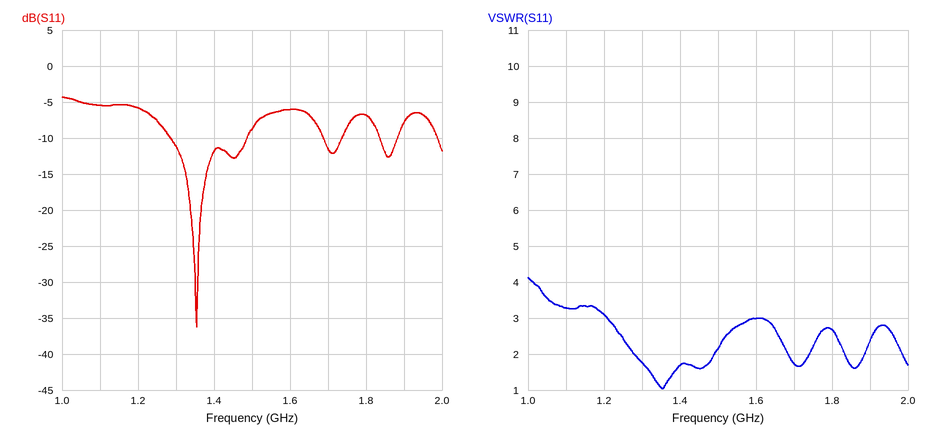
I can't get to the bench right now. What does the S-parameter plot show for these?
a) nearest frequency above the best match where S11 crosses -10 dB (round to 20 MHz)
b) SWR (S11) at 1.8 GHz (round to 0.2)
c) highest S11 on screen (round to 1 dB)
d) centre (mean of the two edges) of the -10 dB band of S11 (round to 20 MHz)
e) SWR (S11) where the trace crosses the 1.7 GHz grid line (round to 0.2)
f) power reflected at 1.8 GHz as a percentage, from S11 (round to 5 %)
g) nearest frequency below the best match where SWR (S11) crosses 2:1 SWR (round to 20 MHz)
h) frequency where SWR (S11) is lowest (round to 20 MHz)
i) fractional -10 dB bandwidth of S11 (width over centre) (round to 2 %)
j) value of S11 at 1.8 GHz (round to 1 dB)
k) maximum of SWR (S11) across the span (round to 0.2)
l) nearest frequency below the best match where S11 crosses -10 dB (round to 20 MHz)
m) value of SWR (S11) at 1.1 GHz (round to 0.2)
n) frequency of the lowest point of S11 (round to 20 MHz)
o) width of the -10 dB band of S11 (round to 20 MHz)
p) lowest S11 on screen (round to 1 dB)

1.48 GHz
2.6
-4 dB
1.38 GHz
1.8
20 %
1.28 GHz
1.36 GHz
14 %
-7 dB
4.2
1.28 GHz
3.2
1.36 GHz
200 MHz
-36 dB
